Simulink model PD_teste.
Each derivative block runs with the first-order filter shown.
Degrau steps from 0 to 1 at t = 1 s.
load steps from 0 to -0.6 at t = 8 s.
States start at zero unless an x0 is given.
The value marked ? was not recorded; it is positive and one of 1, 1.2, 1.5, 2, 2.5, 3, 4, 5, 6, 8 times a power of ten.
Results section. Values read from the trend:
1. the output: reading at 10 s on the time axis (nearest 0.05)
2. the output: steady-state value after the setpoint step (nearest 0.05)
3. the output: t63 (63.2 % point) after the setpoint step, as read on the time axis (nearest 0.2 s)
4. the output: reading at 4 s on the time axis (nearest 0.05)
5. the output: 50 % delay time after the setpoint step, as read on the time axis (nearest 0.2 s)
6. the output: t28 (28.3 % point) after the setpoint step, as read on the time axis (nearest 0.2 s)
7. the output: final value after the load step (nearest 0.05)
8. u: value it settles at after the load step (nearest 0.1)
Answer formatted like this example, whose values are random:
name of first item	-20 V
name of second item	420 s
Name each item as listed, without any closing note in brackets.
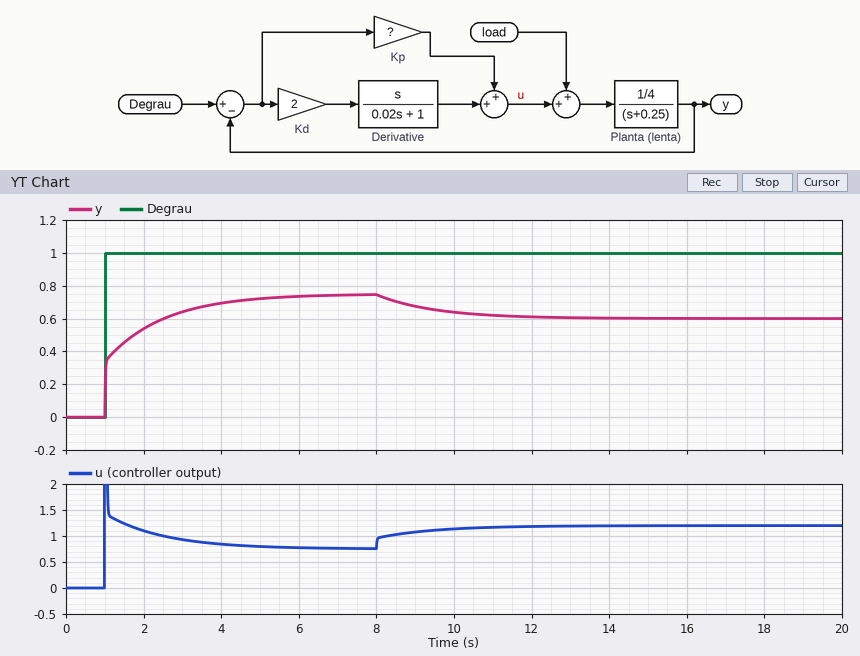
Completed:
the output: reading at 10 s on the time axis	0.65
the output: steady-state value after the setpoint step	0.75
the output: t63 (63.2 % point) after the setpoint step, as read on the time axis	1.6 s
the output: reading at 4 s on the time axis	0.70
the output: 50 % delay time after the setpoint step, as read on the time axis	1.2 s
the output: t28 (28.3 % point) after the setpoint step, as read on the time axis	1.0 s
the output: final value after the load step	0.60
u: value it settles at after the load step	1.2
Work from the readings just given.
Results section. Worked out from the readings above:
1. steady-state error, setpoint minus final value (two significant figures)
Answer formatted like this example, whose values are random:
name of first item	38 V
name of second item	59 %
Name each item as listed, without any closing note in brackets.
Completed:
steady-state error, setpoint minus final value	0.25
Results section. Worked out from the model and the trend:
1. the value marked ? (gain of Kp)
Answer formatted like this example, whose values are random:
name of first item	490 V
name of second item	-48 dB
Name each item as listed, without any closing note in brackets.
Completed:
the value marked ?	3
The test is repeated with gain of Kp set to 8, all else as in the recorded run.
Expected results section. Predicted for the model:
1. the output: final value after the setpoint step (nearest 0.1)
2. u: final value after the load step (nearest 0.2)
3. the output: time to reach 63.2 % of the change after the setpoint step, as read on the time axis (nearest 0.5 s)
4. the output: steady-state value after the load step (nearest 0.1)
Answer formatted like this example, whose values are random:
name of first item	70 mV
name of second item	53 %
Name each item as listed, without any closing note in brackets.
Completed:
the output: final value after the setpoint step	0.9
u: final value after the load step	1.4
the output: time to reach 63.2 % of the change after the setpoint step, as read on the time axis	1.5 s
the output: steady-state value after the load step	0.8
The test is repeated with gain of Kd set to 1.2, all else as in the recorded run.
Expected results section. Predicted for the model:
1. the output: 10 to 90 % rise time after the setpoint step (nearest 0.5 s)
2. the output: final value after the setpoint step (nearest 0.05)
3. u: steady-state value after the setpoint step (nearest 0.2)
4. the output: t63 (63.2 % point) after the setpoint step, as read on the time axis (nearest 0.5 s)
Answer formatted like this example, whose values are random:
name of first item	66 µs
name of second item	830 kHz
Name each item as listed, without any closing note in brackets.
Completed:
the output: 10 to 90 % rise time after the setpoint step	2.5 s
the output: final value after the setpoint step	0.75
u: steady-state value after the setpoint step	0.8
the output: t63 (63.2 % point) after the setpoint step, as read on the time axis	2.0 s
